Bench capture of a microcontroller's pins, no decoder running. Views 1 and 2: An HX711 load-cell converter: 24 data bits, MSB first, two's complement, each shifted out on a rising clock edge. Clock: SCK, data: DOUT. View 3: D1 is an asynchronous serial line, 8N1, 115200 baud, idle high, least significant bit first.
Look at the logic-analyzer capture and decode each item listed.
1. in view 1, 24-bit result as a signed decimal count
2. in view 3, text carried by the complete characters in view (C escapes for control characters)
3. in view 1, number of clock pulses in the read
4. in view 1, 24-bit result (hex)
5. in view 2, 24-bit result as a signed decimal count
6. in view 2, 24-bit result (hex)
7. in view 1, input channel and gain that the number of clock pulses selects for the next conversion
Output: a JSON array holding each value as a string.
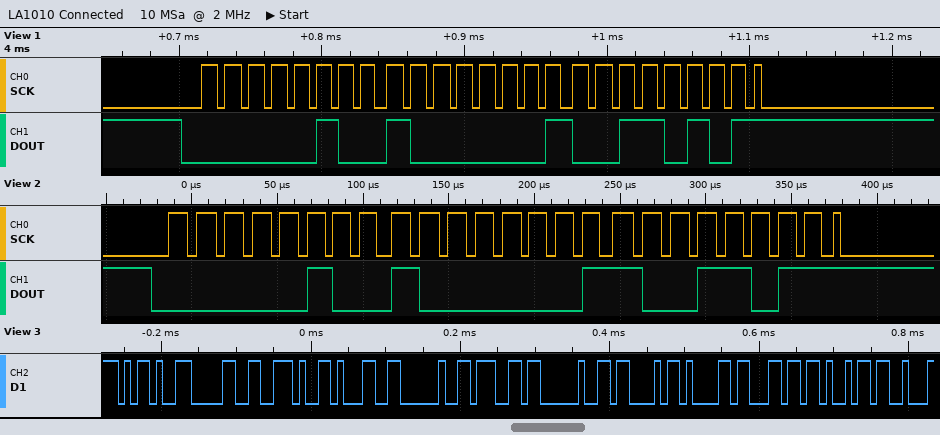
["295221", "\"-0.1 g Cali\"", "25", "0x048135", "295323", "0x04819B", "channel A, gain 128"]
